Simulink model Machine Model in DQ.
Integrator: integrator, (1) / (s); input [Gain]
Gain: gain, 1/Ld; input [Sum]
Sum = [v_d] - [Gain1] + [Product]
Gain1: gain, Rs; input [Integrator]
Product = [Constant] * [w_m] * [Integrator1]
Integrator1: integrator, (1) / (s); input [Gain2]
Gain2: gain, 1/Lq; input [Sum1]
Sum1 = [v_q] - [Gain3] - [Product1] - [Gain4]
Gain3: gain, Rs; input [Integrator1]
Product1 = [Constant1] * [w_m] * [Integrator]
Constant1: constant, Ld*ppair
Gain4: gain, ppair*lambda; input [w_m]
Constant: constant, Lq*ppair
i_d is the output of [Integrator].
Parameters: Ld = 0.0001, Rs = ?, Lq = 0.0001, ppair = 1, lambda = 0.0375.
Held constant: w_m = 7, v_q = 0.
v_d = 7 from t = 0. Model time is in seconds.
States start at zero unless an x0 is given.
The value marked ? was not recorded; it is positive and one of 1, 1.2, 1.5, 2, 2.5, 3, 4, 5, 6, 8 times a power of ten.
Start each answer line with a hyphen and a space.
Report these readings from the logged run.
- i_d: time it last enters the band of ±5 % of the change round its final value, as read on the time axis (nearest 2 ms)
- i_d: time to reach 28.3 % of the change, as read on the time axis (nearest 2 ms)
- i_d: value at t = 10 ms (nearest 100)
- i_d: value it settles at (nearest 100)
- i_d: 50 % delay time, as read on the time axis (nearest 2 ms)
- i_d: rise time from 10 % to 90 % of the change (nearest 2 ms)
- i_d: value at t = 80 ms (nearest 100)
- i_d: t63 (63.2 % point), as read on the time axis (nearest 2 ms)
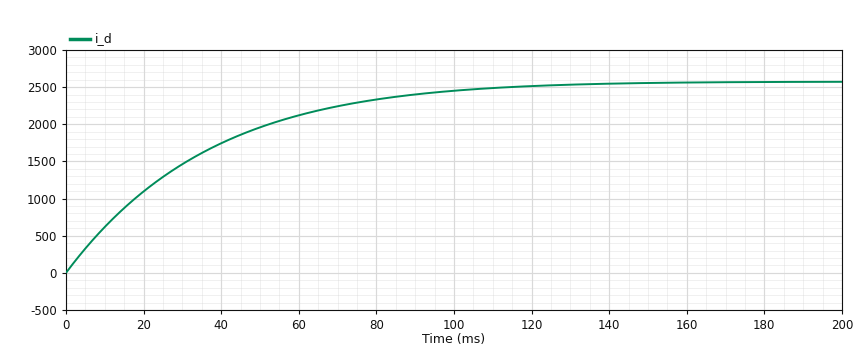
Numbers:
- 98 ms
- 12 ms
- 600
- 2600
- 24 ms
- 74 ms
- 2300
- 36 ms
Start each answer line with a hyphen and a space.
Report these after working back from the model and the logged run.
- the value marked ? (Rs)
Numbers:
- 0.0025
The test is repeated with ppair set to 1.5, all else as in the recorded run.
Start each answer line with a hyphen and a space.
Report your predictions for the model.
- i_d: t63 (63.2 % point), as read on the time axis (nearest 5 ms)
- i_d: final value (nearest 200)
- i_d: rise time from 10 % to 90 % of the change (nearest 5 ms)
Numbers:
- 30 ms
- 2400
- 60 ms
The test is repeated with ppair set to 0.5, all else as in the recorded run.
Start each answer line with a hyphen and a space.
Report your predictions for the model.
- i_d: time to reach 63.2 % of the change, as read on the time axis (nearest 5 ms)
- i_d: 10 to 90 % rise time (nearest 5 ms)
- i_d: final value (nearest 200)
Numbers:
- 40 ms
- 85 ms
- 2800
